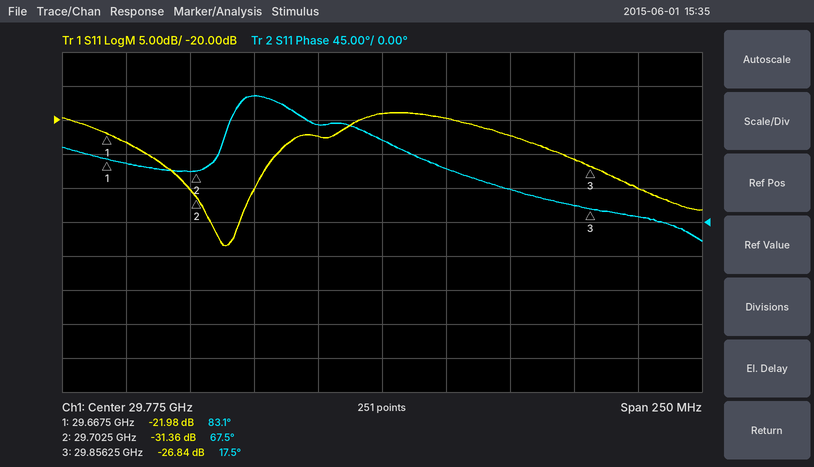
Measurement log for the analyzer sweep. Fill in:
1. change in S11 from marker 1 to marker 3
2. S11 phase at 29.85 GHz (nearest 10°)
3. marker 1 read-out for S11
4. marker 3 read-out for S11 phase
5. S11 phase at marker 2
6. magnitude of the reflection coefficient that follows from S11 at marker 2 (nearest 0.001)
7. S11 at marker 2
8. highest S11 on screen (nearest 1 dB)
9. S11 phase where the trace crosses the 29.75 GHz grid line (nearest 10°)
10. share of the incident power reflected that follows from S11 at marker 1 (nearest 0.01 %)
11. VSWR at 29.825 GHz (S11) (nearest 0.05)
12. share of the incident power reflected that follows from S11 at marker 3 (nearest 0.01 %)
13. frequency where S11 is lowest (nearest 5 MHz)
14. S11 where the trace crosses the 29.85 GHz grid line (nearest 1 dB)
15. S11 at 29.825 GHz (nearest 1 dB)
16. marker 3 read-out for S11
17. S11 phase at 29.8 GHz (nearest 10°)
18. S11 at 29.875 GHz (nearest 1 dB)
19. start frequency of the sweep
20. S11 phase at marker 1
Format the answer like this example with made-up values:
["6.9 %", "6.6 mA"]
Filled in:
["-4.86 dB", "20°", "-21.98 dB", "17.5°", "67.5°", "0.027", "-31.36 dB", "-19 dB", "130°", "0.63 %", "1.15", "0.21 %", "29.715 GHz", "-26 dB", "-22 dB", "-26.84 dB", "70°", "-30 dB", "29.65 GHz", "83.1°"]
